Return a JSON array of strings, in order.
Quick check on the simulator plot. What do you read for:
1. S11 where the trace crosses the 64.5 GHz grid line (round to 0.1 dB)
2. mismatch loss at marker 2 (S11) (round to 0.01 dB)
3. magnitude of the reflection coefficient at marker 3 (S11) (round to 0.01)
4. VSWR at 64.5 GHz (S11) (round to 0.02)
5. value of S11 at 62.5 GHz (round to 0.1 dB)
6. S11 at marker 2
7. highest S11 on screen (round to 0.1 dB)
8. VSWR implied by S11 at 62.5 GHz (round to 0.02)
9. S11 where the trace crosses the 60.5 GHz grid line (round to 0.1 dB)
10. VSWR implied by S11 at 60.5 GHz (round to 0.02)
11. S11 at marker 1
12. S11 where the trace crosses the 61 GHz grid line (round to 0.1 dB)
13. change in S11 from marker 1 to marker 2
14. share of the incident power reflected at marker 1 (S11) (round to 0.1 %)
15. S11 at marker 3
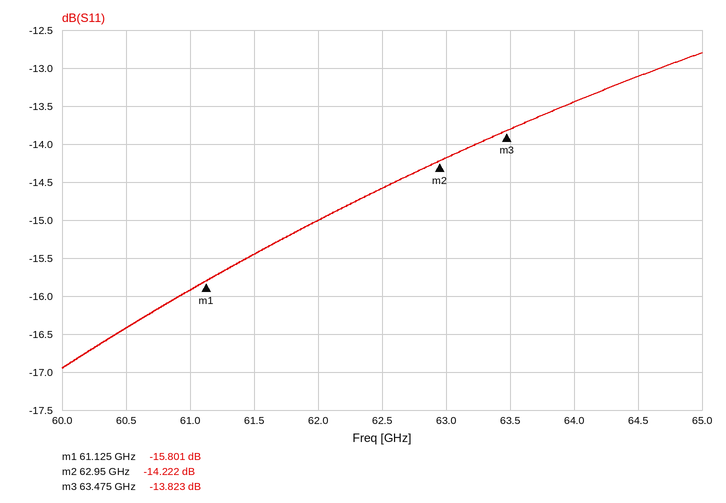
["-13.1 dB", "0.17 dB", "0.20", "1.56", "-14.6 dB", "-14.222 dB", "-12.8 dB", "1.46", "-16.4 dB", "1.36", "-15.801 dB", "-15.9 dB", "1.579 dB", "2.6 %", "-13.823 dB"]
